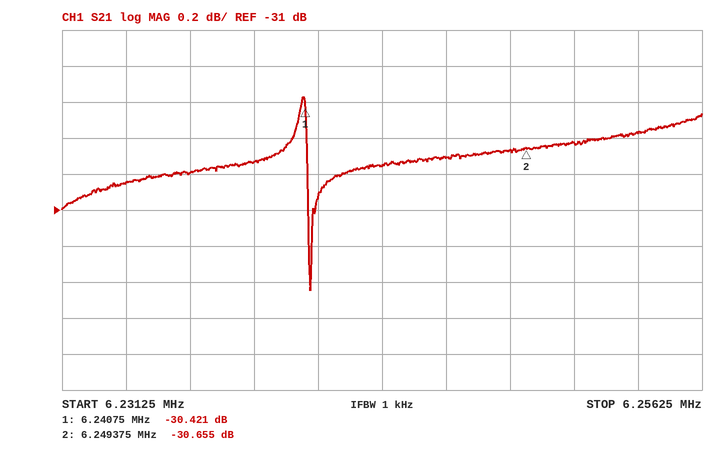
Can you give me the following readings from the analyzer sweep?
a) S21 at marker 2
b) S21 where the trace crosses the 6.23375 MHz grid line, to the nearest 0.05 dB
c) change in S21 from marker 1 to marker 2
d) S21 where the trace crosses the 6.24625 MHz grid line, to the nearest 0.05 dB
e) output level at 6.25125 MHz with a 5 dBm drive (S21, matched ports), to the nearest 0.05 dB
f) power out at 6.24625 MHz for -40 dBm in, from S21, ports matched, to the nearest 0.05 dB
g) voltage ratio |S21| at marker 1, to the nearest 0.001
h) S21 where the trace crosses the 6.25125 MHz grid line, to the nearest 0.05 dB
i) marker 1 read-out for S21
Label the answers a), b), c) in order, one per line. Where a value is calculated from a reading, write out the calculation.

a) -30.655 dB
b) -30.85 dB
c) -30.655 − (-30.421) = -0.234 dB
d) -30.70 dB
e) 5 dBm + (-30.65 dB) = -25.65 dBm
f) -40 dBm + (-30.70 dB) = -70.70 dBm
g) 10^(-30.421/20) ≈ 0.030
h) -30.65 dB
i) -30.421 dB
